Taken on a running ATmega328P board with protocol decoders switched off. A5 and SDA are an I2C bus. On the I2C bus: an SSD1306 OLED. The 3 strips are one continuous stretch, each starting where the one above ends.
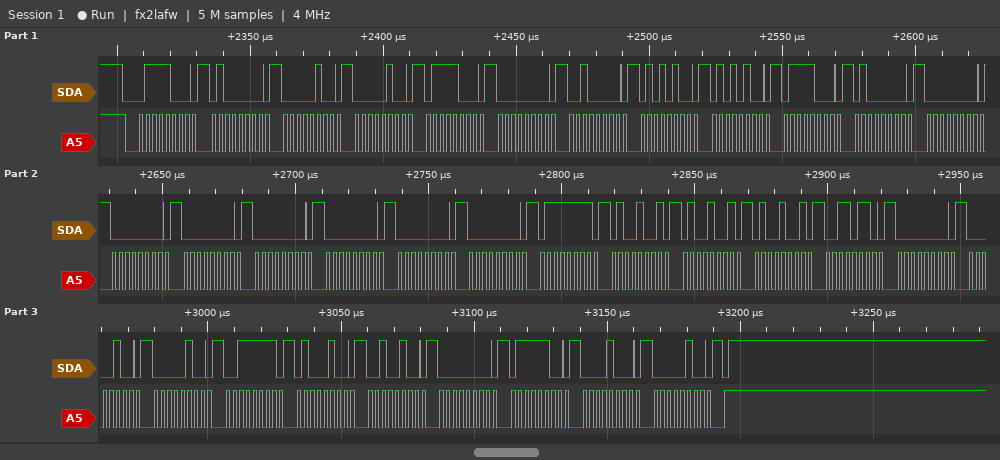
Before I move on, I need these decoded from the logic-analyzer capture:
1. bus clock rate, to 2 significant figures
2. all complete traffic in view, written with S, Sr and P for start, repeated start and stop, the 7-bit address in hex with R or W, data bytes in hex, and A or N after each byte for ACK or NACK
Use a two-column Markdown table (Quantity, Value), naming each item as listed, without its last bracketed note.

| Quantity | Value |
|---|---|
| bus clock rate, to 2 significant figures | 400 kHz |
| all complete traffic in view, written with S, Sr and P for start, repeated start and stop, the 7-bit address in hex with R or W, data bytes in hex, and A or N after each byte for ACK or NACK | S 3CW A 40 A 04 A 04 A 78 A 00 A 20 A 54 A 54 A 78 A 40 A 00 A 00 A 00 A 00 A 00 A 00 A 00 A 7F A 49 A 49 A 49 A 36 A 00 A 04 A 04 A 3F A 44 A 24 A 00 A 7C A 08 A 04 A P |
